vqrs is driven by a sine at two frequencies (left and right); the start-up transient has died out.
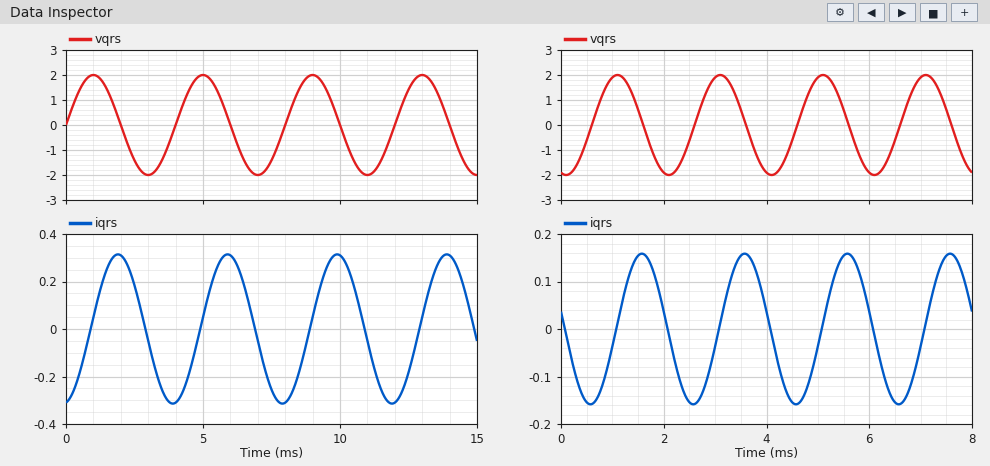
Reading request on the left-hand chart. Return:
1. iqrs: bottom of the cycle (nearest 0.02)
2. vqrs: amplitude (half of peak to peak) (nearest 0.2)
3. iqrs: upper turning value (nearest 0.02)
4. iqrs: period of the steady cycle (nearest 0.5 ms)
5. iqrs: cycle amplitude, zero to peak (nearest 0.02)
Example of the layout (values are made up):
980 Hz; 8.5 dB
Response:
-0.32; 2.0; 0.32; 4.0 ms; 0.32
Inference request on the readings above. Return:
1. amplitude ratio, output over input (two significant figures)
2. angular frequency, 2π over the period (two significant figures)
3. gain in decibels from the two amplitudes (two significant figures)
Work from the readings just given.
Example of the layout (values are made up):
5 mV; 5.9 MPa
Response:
0.16; 1.6 rad/ms; -16 dB
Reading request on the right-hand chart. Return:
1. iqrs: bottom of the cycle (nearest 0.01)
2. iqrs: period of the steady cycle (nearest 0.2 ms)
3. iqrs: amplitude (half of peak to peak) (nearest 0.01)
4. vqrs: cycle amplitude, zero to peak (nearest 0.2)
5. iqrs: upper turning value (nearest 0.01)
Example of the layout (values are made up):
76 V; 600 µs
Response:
-0.16; 2.0 ms; 0.16; 2.0; 0.16
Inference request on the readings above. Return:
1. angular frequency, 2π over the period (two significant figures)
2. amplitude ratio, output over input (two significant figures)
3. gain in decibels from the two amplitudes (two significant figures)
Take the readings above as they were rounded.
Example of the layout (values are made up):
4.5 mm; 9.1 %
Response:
3.1 rad/ms; 0.080; -22 dB
